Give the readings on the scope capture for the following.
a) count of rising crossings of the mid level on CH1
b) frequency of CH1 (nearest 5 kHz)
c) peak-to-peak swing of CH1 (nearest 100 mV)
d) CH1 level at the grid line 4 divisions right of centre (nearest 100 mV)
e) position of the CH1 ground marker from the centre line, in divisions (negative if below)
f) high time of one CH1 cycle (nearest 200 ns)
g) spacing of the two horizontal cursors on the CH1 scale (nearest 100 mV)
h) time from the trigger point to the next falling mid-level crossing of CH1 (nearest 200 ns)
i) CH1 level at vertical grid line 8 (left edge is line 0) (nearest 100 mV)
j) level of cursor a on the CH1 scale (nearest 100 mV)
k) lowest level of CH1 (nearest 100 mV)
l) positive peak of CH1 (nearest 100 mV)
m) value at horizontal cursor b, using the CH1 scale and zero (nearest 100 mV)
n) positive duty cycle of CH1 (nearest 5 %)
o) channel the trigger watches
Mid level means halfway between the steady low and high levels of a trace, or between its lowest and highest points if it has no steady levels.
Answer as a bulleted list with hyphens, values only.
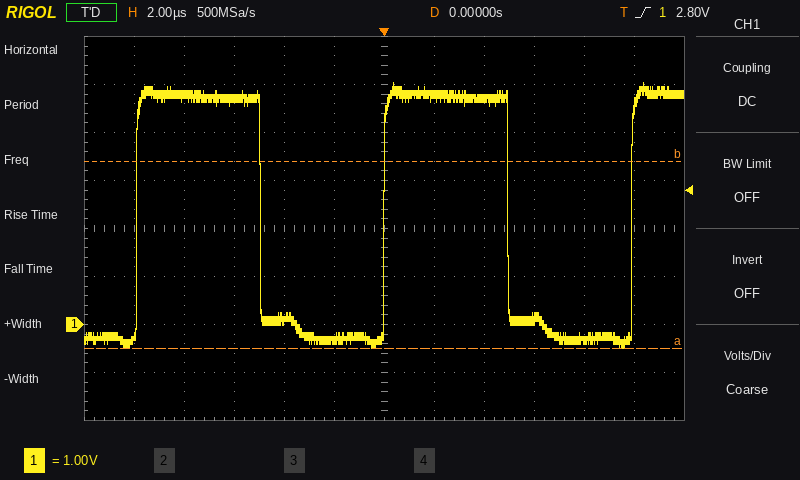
- 3
- 100 kHz
- 5.5 V
- -300 mV
- -2.0 div
- 5.0 µs
- 3.9 V
- 5.0 µs
- 4.7 V
- -500 mV
- -500 mV
- 5.0 V
- 3.4 V
- 50 %
- CH1
